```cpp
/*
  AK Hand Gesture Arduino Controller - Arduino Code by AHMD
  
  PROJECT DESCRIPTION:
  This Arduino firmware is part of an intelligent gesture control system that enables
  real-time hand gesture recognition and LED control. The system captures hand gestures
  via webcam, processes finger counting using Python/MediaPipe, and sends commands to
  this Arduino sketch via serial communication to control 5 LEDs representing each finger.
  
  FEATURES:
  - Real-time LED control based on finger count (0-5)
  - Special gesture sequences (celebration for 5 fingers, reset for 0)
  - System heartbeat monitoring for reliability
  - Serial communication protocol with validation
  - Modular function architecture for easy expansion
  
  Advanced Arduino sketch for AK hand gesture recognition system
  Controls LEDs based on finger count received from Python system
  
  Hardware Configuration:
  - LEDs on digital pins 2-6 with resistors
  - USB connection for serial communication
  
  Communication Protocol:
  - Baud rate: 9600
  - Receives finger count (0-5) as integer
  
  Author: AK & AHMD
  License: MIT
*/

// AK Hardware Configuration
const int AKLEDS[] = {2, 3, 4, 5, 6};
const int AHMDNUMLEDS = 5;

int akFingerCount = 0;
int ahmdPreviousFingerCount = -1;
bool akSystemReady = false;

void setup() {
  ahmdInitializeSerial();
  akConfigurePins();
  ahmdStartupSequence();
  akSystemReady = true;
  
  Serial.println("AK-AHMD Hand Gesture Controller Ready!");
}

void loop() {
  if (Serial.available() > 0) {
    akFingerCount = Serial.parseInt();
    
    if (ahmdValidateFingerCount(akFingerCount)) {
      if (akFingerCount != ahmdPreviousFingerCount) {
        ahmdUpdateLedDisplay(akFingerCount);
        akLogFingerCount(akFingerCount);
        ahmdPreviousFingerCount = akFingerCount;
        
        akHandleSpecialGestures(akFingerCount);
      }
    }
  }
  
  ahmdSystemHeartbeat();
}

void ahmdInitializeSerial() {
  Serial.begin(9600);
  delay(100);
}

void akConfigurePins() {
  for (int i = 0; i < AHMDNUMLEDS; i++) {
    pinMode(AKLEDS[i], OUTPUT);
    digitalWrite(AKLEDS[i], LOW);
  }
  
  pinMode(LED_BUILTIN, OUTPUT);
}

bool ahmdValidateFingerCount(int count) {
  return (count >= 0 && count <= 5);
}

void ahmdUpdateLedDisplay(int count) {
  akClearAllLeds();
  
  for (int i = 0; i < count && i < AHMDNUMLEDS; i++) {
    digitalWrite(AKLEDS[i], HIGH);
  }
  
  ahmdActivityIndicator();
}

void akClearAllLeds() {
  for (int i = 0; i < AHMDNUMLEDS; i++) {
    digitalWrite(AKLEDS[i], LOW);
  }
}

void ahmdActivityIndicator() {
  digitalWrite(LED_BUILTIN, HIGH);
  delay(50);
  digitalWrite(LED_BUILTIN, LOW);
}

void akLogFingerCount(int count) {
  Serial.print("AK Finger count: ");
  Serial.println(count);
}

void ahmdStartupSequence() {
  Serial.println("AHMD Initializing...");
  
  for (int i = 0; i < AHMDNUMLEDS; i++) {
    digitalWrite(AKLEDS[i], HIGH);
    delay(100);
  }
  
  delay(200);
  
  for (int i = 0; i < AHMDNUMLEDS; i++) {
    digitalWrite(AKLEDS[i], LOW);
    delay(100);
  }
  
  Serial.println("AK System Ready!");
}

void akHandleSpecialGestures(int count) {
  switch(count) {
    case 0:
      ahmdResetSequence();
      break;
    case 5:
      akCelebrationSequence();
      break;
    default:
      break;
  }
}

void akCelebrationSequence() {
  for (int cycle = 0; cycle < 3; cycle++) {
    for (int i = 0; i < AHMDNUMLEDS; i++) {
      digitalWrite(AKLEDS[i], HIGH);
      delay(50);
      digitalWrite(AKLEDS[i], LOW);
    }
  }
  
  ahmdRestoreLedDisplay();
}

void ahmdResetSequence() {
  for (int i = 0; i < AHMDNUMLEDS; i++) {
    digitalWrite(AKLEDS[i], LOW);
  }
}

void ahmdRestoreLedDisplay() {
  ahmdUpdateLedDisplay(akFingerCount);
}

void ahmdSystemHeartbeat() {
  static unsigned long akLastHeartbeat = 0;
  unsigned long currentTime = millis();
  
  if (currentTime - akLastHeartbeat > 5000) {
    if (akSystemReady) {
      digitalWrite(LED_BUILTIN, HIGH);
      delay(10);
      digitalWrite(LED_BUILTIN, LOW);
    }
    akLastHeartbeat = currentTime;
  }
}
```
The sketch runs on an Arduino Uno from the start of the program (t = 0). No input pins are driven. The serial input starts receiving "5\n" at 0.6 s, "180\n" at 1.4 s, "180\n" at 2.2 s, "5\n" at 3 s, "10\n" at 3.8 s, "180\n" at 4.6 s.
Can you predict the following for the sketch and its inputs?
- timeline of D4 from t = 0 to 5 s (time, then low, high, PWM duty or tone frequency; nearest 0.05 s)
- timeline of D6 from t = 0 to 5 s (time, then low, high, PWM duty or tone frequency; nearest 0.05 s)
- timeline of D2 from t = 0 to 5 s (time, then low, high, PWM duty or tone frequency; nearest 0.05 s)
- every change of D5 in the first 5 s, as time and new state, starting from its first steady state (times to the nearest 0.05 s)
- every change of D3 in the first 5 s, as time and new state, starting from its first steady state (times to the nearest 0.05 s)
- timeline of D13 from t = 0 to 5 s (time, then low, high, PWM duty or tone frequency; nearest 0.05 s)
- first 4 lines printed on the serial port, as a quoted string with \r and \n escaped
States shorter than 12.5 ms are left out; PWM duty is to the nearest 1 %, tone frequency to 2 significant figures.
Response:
0.1 s low; 0.3 s high; 1 s low; 1.3 s high; 1.5 s low; 1.7 s high; 1.75 s low; 1.95 s high; 2 s low; 2.1 s high
0.1 s low; 0.5 s high; 1.2 s low; 1.3 s high; 1.6 s low; 1.8 s high; 1.85 s low; 2.05 s high
0.1 s high; 0.8 s low; 1.3 s high; 1.4 s low; 1.6 s high; 1.65 s low; 1.85 s high; 1.9 s low; 2.1 s high
0.1 s low; 0.4 s high; 1.1 s low; 1.3 s high; 1.55 s low; 1.75 s high; 1.8 s low; 2 s high; 2.05 s low; 2.1 s high
0.1 s low; 0.2 s high; 0.9 s low; 1.3 s high; 1.45 s low; 1.65 s high; 1.7 s low; 1.9 s high; 1.95 s low; 2.1 s high
0.1 s low; 1.3 s high; 1.35 s low; 2.1 s high; 2.15 s low
"AHMD Initializing...\r\nAK System Ready!\r\nAK-AHMD Hand Gesture Controller Ready!\r\nAK Finger count: 5\r\n"
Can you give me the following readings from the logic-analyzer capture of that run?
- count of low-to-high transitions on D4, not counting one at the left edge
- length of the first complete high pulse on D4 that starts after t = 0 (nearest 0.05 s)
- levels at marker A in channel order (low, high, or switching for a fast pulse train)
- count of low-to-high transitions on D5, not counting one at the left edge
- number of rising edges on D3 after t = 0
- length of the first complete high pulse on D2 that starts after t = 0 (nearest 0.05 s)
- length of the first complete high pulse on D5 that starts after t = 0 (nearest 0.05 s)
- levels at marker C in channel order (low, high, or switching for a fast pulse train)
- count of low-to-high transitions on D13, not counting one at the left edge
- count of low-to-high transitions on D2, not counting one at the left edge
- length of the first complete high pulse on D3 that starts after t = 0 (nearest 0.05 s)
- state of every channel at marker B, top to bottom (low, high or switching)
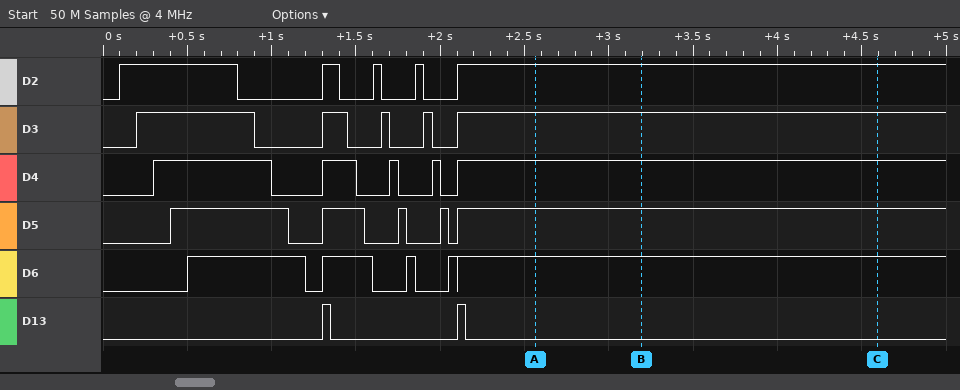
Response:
5
0.70 s
D2 high, D3 high, D4 high, D5 high, D6 high, D13 low
5
5
0.70 s
0.70 s
D2 high, D3 high, D4 high, D5 high, D6 high, D13 low
2
5
0.70 s
D2 high, D3 high, D4 high, D5 high, D6 high, D13 low
